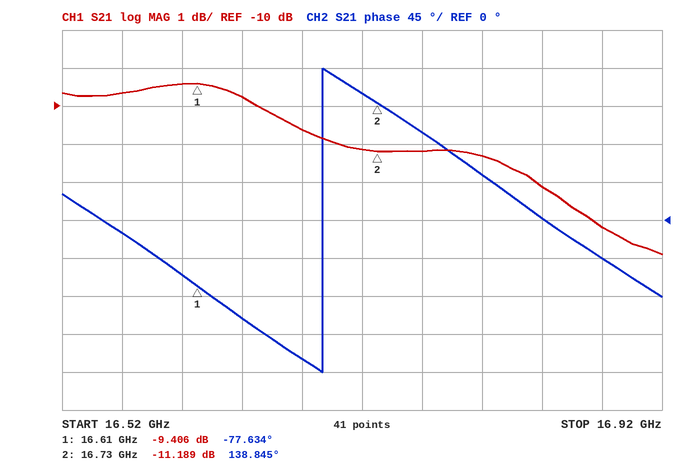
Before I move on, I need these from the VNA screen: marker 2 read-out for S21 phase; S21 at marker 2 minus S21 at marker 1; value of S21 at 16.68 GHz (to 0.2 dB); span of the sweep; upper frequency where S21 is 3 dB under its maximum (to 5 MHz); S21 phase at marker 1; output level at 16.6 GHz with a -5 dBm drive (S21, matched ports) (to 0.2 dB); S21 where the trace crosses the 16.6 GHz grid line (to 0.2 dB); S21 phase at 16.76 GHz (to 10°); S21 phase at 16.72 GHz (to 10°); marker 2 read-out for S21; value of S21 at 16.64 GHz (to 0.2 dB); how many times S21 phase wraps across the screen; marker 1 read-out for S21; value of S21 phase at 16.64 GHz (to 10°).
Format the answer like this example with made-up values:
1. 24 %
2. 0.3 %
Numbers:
1. 138.845°
2. -1.783 dB
3. -10.6 dB
4. 400 MHz
5. 16.850 GHz
6. -77.634°
7. -14.4 dBm
8. -9.4 dB
9. 100°
10. 150°
11. -11.189 dB
12. -9.8 dB
13. 1
14. -9.406 dB
15. -120°
